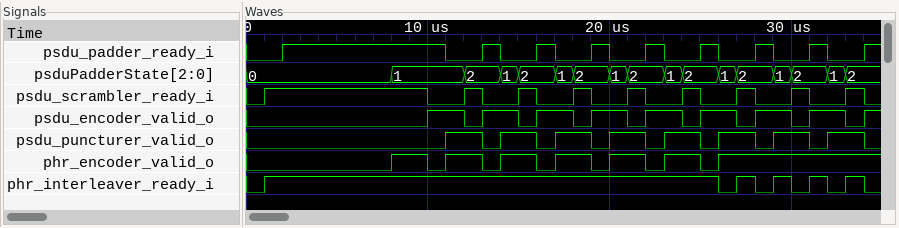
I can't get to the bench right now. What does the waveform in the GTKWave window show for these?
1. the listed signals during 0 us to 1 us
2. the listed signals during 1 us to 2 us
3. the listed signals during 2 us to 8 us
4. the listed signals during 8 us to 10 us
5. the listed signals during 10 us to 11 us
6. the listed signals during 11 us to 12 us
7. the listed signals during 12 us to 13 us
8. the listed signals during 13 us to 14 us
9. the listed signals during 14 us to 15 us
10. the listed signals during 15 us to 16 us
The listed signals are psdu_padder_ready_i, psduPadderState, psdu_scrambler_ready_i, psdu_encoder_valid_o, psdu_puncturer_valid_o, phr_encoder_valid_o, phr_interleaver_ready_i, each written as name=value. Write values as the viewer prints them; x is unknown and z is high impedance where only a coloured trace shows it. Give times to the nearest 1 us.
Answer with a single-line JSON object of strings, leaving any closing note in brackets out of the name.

{"the listed signals during 0 us to 1 us": "psdu_padder_ready_i=0, psduPadderState=0, psdu_scrambler_ready_i=0, psdu_encoder_valid_o=0, psdu_puncturer_valid_o=0, phr_encoder_valid_o=0, phr_interleaver_ready_i=0", "the listed signals during 1 us to 2 us": "psdu_padder_ready_i=0, psduPadderState=0, psdu_scrambler_ready_i=1, psdu_encoder_valid_o=0, psdu_puncturer_valid_o=0, phr_encoder_valid_o=0, phr_interleaver_ready_i=1", "the listed signals during 2 us to 8 us": "psdu_padder_ready_i=1, psduPadderState=0, psdu_scrambler_ready_i=1, psdu_encoder_valid_o=0, psdu_puncturer_valid_o=0, phr_encoder_valid_o=0, phr_interleaver_ready_i=1", "the listed signals during 8 us to 10 us": "psdu_padder_ready_i=1, psduPadderState=1, psdu_scrambler_ready_i=1, psdu_encoder_valid_o=0, psdu_puncturer_valid_o=0, phr_encoder_valid_o=1, phr_interleaver_ready_i=1", "the listed signals during 10 us to 11 us": "psdu_padder_ready_i=1, psduPadderState=1, psdu_scrambler_ready_i=0, psdu_encoder_valid_o=1, psdu_puncturer_valid_o=0, phr_encoder_valid_o=0, phr_interleaver_ready_i=1", "the listed signals during 11 us to 12 us": "psdu_padder_ready_i=0, psduPadderState=1, psdu_scrambler_ready_i=0, psdu_encoder_valid_o=1, psdu_puncturer_valid_o=1, phr_encoder_valid_o=1, phr_interleaver_ready_i=1", "the listed signals during 12 us to 13 us": "psdu_padder_ready_i=0, psduPadderState=2, psdu_scrambler_ready_i=1, psdu_encoder_valid_o=0, psdu_puncturer_valid_o=1, phr_encoder_valid_o=1, phr_interleaver_ready_i=1", "the listed signals during 13 us to 14 us": "psdu_padder_ready_i=1, psduPadderState=2, psdu_scrambler_ready_i=0, psdu_encoder_valid_o=1, psdu_puncturer_valid_o=0, phr_encoder_valid_o=0, phr_interleaver_ready_i=1", "the listed signals during 14 us to 15 us": "psdu_padder_ready_i=0, psduPadderState=1, psdu_scrambler_ready_i=0, psdu_encoder_valid_o=1, psdu_puncturer_valid_o=1, phr_encoder_valid_o=1, phr_interleaver_ready_i=1", "the listed signals during 15 us to 16 us": "psdu_padder_ready_i=0, psduPadderState=2, psdu_scrambler_ready_i=1, psdu_encoder_valid_o=0, psdu_puncturer_valid_o=1, phr_encoder_valid_o=1, phr_interleaver_ready_i=1"}
